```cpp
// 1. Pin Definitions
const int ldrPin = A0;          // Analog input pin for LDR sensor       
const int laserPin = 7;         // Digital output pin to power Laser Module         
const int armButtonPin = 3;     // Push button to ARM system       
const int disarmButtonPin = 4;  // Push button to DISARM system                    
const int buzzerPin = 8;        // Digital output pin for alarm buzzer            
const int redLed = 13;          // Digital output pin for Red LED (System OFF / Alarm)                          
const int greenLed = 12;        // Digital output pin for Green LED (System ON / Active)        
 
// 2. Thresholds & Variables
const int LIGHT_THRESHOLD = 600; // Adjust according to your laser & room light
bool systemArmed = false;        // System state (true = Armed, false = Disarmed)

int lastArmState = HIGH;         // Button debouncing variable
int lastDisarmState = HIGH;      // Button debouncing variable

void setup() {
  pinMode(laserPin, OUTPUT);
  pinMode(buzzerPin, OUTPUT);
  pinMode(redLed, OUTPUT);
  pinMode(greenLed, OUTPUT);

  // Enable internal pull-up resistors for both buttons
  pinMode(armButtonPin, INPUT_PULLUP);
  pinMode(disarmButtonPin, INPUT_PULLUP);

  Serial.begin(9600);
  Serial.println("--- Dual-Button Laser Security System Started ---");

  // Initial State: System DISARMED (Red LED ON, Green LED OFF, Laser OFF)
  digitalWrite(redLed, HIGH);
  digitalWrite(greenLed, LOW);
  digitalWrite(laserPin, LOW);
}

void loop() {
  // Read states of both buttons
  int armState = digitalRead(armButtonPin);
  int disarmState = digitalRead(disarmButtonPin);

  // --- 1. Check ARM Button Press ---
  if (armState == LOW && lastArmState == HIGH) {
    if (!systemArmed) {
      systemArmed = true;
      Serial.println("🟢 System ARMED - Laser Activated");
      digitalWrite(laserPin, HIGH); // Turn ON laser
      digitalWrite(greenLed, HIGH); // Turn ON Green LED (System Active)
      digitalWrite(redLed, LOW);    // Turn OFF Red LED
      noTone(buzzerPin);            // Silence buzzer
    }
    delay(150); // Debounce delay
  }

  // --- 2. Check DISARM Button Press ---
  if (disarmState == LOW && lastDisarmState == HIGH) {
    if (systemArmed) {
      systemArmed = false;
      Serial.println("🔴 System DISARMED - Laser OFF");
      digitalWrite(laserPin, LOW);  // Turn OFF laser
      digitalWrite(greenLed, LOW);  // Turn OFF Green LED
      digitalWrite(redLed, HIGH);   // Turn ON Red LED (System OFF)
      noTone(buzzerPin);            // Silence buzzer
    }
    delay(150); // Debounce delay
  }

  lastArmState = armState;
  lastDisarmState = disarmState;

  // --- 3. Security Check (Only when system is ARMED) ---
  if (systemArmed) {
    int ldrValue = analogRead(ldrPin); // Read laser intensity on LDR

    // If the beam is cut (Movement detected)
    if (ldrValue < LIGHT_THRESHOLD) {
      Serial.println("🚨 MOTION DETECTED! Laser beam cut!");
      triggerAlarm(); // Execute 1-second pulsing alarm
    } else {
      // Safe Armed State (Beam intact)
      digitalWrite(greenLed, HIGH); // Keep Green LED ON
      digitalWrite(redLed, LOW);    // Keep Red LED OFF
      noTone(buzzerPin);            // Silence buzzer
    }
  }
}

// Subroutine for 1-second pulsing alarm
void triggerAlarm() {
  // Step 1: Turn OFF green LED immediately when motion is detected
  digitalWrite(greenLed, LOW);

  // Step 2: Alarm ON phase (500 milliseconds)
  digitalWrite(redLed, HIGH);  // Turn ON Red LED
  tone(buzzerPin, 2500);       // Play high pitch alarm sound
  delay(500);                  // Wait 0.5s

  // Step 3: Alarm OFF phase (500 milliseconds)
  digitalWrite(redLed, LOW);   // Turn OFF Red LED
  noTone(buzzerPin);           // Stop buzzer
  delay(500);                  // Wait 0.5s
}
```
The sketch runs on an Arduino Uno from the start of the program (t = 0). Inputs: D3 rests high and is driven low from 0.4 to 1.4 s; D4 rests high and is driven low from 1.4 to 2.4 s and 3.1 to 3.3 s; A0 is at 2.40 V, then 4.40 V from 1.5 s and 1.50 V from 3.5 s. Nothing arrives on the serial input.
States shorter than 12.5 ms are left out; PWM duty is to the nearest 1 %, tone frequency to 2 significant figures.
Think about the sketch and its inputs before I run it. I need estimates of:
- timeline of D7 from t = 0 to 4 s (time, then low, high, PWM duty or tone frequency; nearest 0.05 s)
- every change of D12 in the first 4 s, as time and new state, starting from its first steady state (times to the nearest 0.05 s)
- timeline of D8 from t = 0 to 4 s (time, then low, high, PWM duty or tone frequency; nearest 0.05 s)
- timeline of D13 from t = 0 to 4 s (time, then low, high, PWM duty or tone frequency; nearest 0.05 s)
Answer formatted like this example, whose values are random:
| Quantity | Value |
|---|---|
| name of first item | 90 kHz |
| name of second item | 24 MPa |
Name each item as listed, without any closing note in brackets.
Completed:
| Quantity | Value |
|---|---|
| timeline of D7 from t = 0 to 4 s | 0 s low; 0.4 s high; 1.55 s low |
| every change of D12 in the first 4 s, as time and new state, starting from its first steady state | 0 s low; 0.4 s high; 0.55 s low |
| timeline of D8 from t = 0 to 4 s | 0 s low; 0.55 s tone 2500 Hz; 1.05 s low |
| timeline of D13 from t = 0 to 4 s | 0 s high; 0.4 s low; 0.55 s high; 1.05 s low; 1.55 s high |
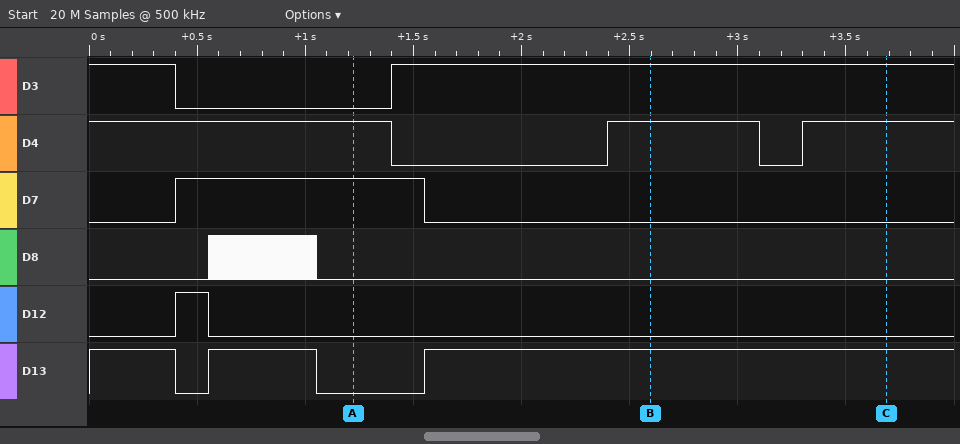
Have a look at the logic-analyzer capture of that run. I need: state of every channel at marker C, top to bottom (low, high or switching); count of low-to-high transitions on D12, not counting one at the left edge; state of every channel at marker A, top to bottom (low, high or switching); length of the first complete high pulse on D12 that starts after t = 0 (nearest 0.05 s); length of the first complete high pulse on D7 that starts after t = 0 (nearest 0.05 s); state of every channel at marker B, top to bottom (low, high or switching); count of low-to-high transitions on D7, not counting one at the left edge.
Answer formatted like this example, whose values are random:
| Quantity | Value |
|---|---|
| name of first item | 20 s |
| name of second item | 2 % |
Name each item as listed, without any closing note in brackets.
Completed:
| Quantity | Value |
|---|---|
| state of every channel at marker C, top to bottom | D3 high, D4 high, D7 low, D8 low, D12 low, D13 high |
| count of low-to-high transitions on D12, not counting one at the left edge | 1 |
| state of every channel at marker A, top to bottom | D3 low, D4 high, D7 high, D8 low, D12 low, D13 low |
| length of the first complete high pulse on D12 that starts after t = 0 | 0.15 s |
| length of the first complete high pulse on D7 that starts after t = 0 | 1.15 s |
| state of every channel at marker B, top to bottom | D3 high, D4 high, D7 low, D8 low, D12 low, D13 high |
| count of low-to-high transitions on D7, not counting one at the left edge | 1 |
